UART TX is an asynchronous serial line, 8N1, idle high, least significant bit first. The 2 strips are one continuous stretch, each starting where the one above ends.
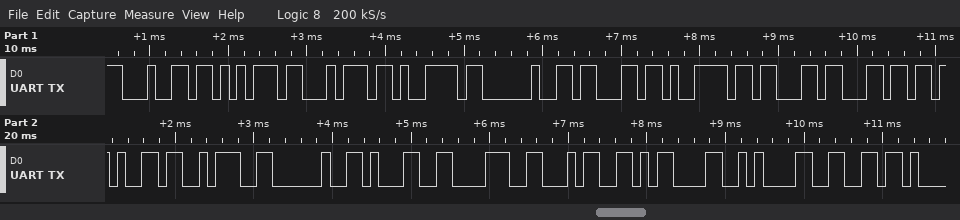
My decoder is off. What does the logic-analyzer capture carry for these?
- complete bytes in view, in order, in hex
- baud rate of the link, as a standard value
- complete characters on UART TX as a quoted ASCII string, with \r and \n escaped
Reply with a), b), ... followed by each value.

a) 0x64 0x75 0x74 0x79 0x20 0x63 0x79 0x63 0x6C 0x65 0x3A 0x20 0x31 0x38 0x34 0x0D 0x0A 0x66
b) 9600 baud
c) "duty cycle: 184\r\nf"
